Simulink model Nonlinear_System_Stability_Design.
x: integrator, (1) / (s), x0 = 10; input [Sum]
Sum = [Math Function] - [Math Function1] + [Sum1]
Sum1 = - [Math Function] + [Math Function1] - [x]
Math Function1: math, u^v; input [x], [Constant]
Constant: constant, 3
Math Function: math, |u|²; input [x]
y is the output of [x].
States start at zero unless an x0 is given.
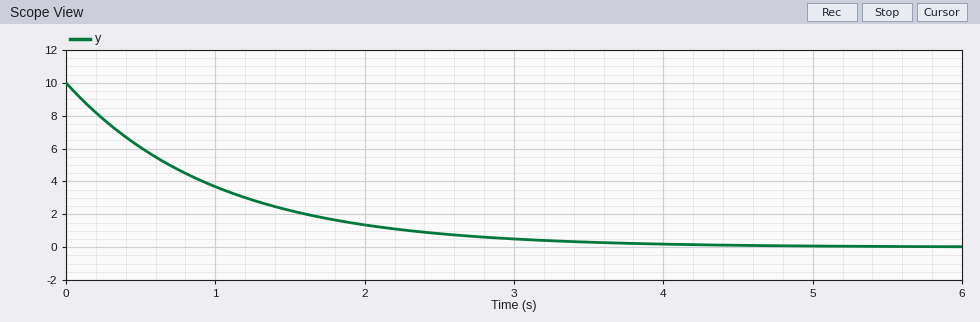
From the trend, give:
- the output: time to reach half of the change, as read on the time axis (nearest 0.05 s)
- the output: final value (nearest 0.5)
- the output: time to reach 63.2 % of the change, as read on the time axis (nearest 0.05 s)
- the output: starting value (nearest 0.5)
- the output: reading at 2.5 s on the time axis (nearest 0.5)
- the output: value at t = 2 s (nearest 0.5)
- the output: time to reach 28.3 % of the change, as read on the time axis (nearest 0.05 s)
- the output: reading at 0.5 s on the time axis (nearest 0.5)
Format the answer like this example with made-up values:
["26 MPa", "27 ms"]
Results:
["0.70 s", "0.0", "1.00 s", "10.0", "1.0", "1.5", "0.35 s", "6.0"]
